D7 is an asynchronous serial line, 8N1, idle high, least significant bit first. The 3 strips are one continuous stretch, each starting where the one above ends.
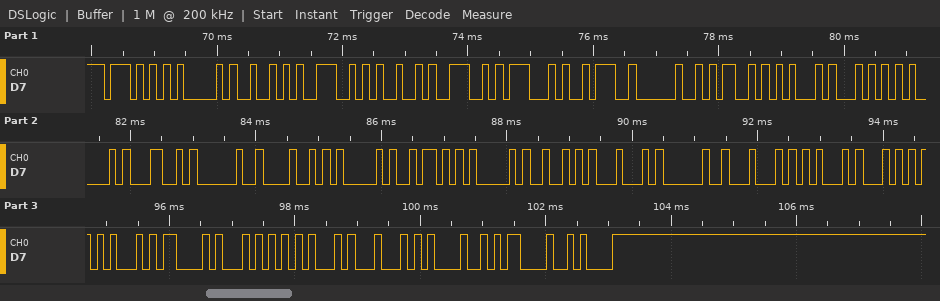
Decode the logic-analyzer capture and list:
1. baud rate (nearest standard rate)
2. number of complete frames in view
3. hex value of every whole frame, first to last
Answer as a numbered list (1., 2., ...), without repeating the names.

1. 9600 baud
2. 33
3. 57 41 52 4E 49 4E 47 3A 20 4D 45 54 41 4C 20 48 41 5A 41 52 44 20 44 45 54 45 43 54 45 44 21 0D 0A
